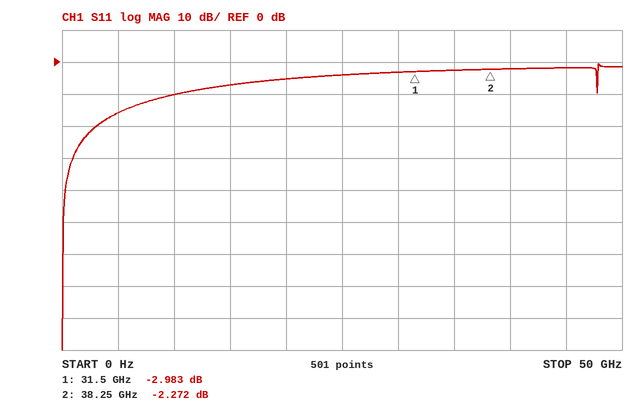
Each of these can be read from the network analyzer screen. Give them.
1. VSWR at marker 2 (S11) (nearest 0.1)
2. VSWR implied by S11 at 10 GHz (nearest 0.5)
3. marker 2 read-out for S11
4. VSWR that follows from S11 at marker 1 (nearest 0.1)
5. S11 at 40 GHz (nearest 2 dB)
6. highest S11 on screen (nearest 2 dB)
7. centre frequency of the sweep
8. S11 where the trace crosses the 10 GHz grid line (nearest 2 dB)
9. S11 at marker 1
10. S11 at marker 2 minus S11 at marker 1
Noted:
7.7
2.0
-2.272 dB
5.9
-2 dB
0 dB
25 GHz
-10 dB
-2.983 dB
0.711 dB
